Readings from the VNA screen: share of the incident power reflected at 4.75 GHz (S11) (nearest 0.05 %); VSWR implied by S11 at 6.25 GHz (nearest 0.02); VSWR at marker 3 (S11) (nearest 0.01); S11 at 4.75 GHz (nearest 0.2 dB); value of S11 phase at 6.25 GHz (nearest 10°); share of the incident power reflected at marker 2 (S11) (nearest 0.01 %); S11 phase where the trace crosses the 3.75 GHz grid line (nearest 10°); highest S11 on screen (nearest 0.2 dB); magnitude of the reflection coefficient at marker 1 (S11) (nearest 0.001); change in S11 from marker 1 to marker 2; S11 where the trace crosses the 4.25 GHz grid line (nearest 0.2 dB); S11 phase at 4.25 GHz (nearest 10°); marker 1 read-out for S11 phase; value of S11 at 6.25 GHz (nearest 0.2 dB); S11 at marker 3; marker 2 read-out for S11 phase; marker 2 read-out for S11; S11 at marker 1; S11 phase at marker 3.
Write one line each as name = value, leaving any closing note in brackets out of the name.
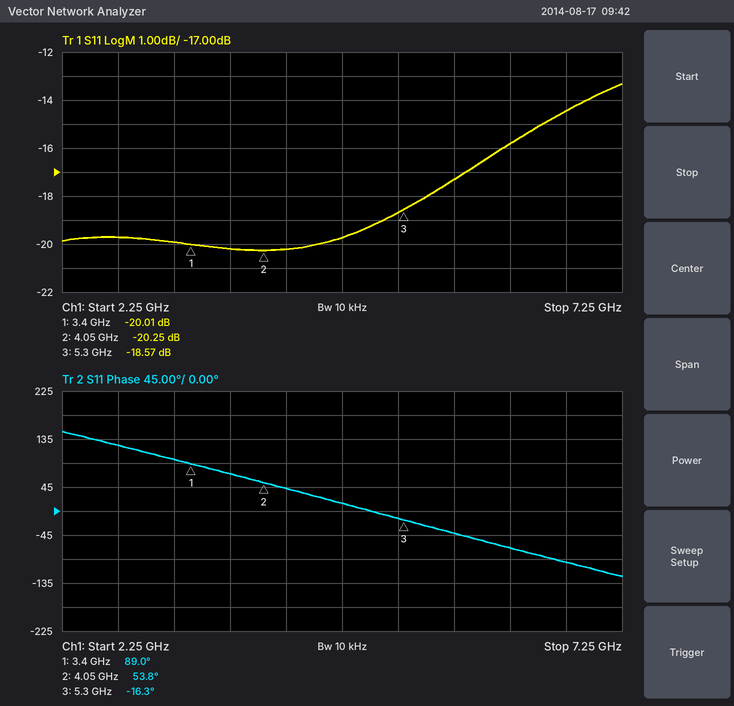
share of the incident power reflected at 4.75 GHz (S11) = 1.05 %
VSWR implied by S11 at 6.25 GHz = 1.38
VSWR at marker 3 (S11) = 1.27
S11 at 4.75 GHz = -19.8 dB
value of S11 phase at 6.25 GHz = -70°
share of the incident power reflected at marker 2 (S11) = 0.94 %
S11 phase where the trace crosses the 3.75 GHz grid line = 70°
highest S11 on screen = -13.4 dB
magnitude of the reflection coefficient at marker 1 (S11) = 0.100
change in S11 from marker 1 to marker 2 = -0.24 dB
S11 where the trace crosses the 4.25 GHz grid line = -20.2 dB
S11 phase at 4.25 GHz = 40°
marker 1 read-out for S11 phase = 89.0°
value of S11 at 6.25 GHz = -15.8 dB
S11 at marker 3 = -18.57 dB
marker 2 read-out for S11 phase = 53.8°
marker 2 read-out for S11 = -20.25 dB
S11 at marker 1 = -20.01 dB
S11 phase at marker 3 = -16.3°
